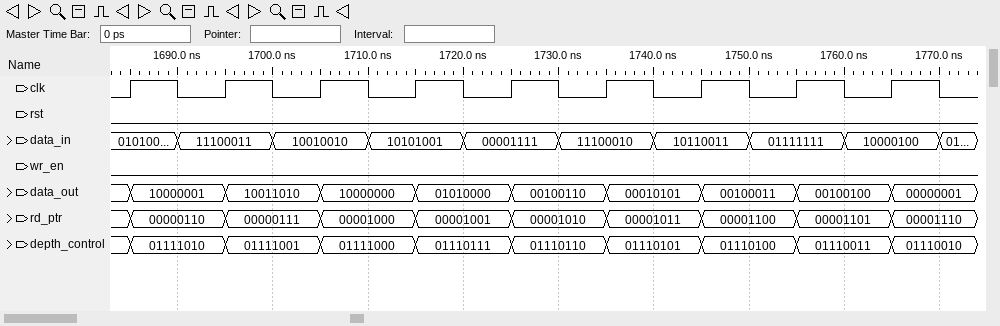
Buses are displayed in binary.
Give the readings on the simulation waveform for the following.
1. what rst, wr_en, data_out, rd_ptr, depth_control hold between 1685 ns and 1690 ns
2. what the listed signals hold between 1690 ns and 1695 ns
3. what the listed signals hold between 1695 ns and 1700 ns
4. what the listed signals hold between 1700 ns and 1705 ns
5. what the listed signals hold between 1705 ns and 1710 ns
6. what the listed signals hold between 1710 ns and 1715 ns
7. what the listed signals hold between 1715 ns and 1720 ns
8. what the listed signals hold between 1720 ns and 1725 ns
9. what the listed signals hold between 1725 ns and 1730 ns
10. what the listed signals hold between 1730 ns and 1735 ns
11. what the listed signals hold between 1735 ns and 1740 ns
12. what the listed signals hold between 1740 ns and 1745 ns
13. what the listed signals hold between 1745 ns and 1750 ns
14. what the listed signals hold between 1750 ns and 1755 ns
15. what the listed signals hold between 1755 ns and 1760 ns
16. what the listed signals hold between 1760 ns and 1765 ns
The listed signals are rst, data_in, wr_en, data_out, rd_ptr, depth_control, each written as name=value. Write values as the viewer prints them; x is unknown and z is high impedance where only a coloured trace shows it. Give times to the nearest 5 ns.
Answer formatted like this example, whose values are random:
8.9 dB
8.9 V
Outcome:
rst=0, wr_en=0, data_out=10000001, rd_ptr=00000110, depth_control=01111010
rst=0, data_in=11100011, wr_en=0, data_out=10000001, rd_ptr=00000110, depth_control=01111010
rst=0, data_in=11100011, wr_en=0, data_out=10011010, rd_ptr=00000111, depth_control=01111001
rst=0, data_in=10010010, wr_en=0, data_out=10011010, rd_ptr=00000111, depth_control=01111001
rst=0, data_in=10010010, wr_en=0, data_out=10000000, rd_ptr=00001000, depth_control=01111000
rst=0, data_in=10101001, wr_en=0, data_out=10000000, rd_ptr=00001000, depth_control=01111000
rst=0, data_in=10101001, wr_en=0, data_out=01010000, rd_ptr=00001001, depth_control=01110111
rst=0, data_in=00001111, wr_en=0, data_out=01010000, rd_ptr=00001001, depth_control=01110111
rst=0, data_in=00001111, wr_en=0, data_out=00100110, rd_ptr=00001010, depth_control=01110110
rst=0, data_in=11100010, wr_en=0, data_out=00100110, rd_ptr=00001010, depth_control=01110110
rst=0, data_in=11100010, wr_en=0, data_out=00010101, rd_ptr=00001011, depth_control=01110101
rst=0, data_in=10110011, wr_en=0, data_out=00010101, rd_ptr=00001011, depth_control=01110101
rst=0, data_in=10110011, wr_en=0, data_out=00100011, rd_ptr=00001100, depth_control=01110100
rst=0, data_in=01111111, wr_en=0, data_out=00100011, rd_ptr=00001100, depth_control=01110100
rst=0, data_in=01111111, wr_en=0, data_out=00100100, rd_ptr=00001101, depth_control=01110011
rst=0, data_in=10000100, wr_en=0, data_out=00100100, rd_ptr=00001101, depth_control=01110011
